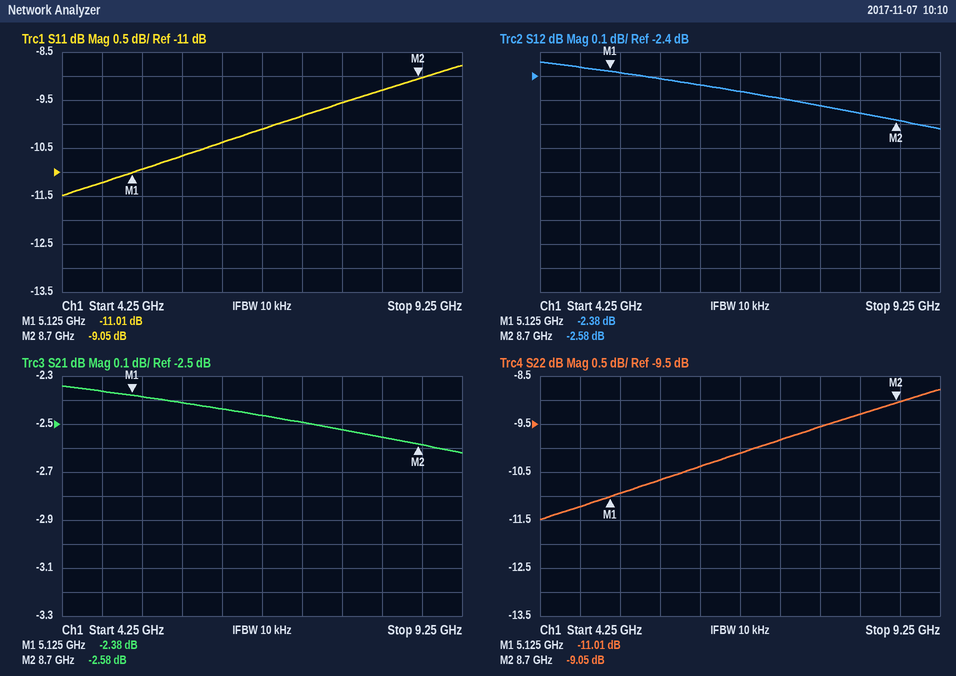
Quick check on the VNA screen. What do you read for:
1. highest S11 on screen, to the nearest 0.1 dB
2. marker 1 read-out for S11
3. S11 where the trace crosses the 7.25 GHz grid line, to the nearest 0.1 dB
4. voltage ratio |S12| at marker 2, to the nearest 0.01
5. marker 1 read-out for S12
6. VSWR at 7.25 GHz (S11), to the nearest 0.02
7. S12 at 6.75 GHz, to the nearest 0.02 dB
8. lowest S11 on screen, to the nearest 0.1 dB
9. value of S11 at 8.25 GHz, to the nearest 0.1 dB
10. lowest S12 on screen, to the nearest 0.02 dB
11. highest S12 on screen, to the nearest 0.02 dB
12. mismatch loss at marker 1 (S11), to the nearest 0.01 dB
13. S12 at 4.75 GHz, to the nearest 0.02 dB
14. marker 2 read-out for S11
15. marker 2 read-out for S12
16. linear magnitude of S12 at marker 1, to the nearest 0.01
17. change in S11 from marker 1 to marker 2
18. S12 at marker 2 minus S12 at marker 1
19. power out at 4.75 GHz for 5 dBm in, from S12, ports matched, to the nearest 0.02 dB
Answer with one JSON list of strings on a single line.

["-8.8 dB", "-11.01 dB", "-9.8 dB", "0.74", "-2.38 dB", "1.96", "-2.46 dB", "-11.5 dB", "-9.3 dB", "-2.62 dB", "-2.34 dB", "0.36 dB", "-2.36 dB", "-9.05 dB", "-2.58 dB", "0.76", "1.96 dB", "-0.20 dB", "2.64 dBm"]
